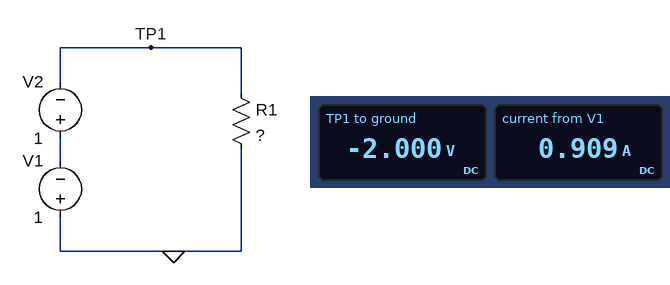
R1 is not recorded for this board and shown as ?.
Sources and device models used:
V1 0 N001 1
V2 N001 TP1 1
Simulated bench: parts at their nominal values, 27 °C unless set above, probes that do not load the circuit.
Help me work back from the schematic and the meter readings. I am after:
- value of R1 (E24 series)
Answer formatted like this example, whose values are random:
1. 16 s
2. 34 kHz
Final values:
1. 2.2 Ω
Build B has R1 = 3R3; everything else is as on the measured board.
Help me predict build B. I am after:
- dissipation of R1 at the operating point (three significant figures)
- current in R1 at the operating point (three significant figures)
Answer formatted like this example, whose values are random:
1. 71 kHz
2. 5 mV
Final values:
1. 1.21 W
2. 606 mA
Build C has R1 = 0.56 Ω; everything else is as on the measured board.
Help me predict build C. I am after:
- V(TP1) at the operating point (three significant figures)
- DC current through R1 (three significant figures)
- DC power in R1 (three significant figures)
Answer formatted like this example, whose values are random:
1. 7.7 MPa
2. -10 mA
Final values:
1. -2.00 V
2. 3.57 A
3. 7.14 W
